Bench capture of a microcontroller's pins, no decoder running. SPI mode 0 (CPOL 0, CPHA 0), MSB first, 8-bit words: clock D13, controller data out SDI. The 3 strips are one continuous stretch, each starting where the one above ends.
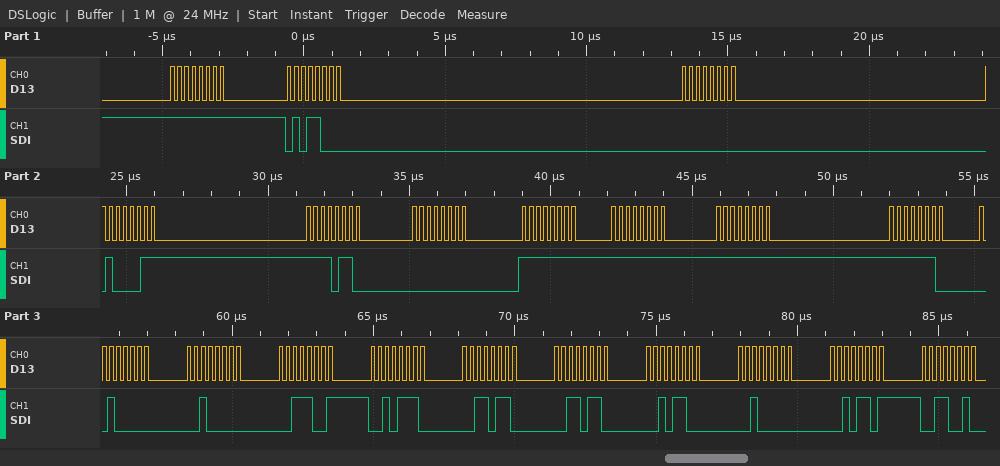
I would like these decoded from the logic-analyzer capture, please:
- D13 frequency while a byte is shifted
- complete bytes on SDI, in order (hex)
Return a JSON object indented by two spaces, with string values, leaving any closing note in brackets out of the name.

{
  "D13 frequency while a byte is shifted": "4 MHz",
  "complete bytes on SDI, in order": "FF 58 00 43 F6 00 FF FF FF FE 20 20 39 2E 36 36 2C 20 2D 32"
}
